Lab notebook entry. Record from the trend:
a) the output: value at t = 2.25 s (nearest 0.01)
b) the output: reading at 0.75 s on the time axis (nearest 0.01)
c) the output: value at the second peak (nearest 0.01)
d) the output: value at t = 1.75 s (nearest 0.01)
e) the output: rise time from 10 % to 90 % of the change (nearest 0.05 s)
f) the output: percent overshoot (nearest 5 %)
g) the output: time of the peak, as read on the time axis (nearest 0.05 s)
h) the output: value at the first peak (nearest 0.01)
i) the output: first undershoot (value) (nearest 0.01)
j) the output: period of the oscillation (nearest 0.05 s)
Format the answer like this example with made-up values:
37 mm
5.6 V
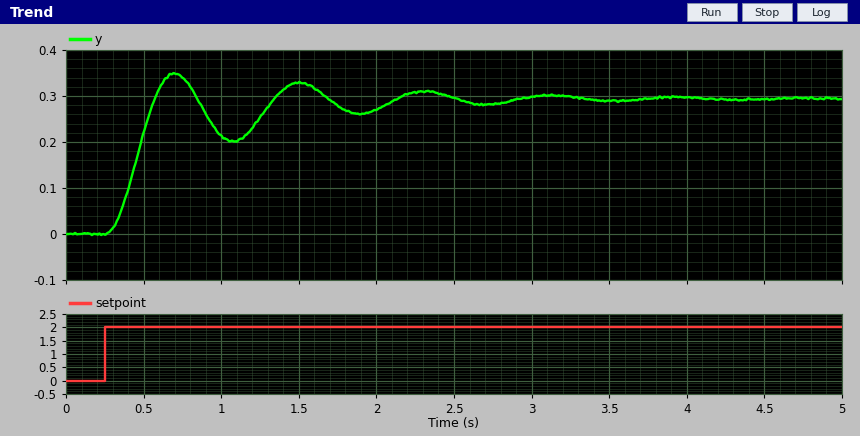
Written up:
0.31
0.34
0.33
0.28
0.20 s
20 %
0.70 s
0.35
0.20
0.80 s
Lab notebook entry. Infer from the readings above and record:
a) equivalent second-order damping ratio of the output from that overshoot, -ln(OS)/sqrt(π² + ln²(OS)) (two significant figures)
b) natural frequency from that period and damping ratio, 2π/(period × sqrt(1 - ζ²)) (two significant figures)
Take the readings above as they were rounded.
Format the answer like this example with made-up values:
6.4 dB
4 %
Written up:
0.46
8.8 rad/s
